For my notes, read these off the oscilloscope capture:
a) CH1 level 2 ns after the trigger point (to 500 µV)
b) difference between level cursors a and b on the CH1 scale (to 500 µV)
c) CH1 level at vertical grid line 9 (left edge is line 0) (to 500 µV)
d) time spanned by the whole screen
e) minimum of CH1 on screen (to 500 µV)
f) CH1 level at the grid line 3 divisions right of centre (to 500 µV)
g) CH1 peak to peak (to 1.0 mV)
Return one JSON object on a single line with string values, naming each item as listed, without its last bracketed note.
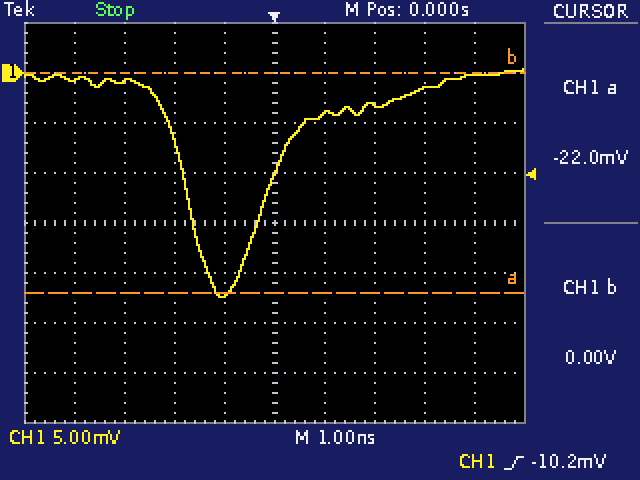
{"CH1 level 2 ns after the trigger point": "-3.0 mV", "difference between level cursors a and b on the CH1 scale": "22.0 mV", "CH1 level at vertical grid line 9 (left edge is line 0)": "0.0 mV", "time spanned by the whole screen": "10 ns", "minimum of CH1 on screen": "-22.5 mV", "CH1 level at the grid line 3 divisions right of centre": "-1.5 mV", "CH1 peak to peak": "23.0 mV"}
